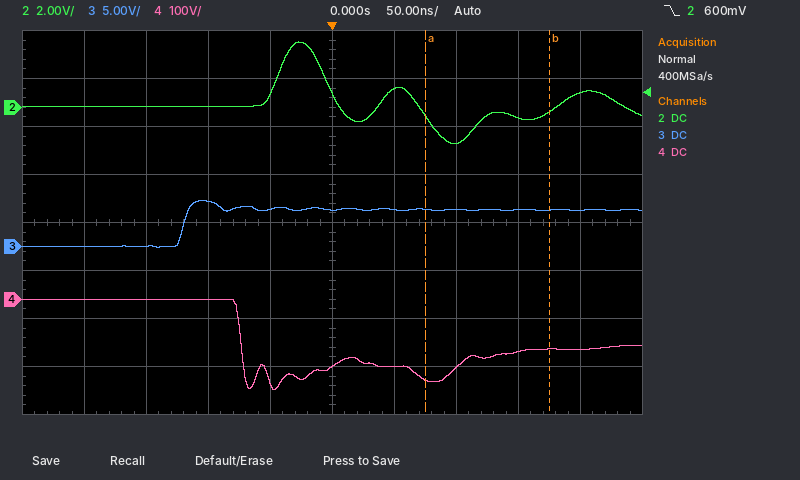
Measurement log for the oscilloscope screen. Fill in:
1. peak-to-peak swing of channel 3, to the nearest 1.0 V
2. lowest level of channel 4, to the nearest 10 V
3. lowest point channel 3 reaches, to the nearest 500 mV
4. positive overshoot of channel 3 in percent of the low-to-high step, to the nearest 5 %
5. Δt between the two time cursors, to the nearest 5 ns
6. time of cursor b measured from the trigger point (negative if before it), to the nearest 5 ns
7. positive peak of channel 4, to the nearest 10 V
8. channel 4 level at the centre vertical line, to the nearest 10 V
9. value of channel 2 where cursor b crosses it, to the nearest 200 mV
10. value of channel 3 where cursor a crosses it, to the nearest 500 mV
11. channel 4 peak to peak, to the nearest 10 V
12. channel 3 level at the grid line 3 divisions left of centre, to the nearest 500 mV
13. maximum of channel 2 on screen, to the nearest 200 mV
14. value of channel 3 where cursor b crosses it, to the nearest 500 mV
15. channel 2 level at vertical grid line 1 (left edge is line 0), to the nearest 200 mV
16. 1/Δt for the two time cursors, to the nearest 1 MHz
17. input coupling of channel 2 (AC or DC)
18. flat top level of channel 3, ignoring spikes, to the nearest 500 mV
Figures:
5.0 V
-190 V
0.0 V
25 %
100 ns
+175 ns
0 V
-140 V
-200 mV
4.0 V
190 V
0.0 V
2.8 V
4.0 V
0.0 V
10 MHz
DC
4.0 V
